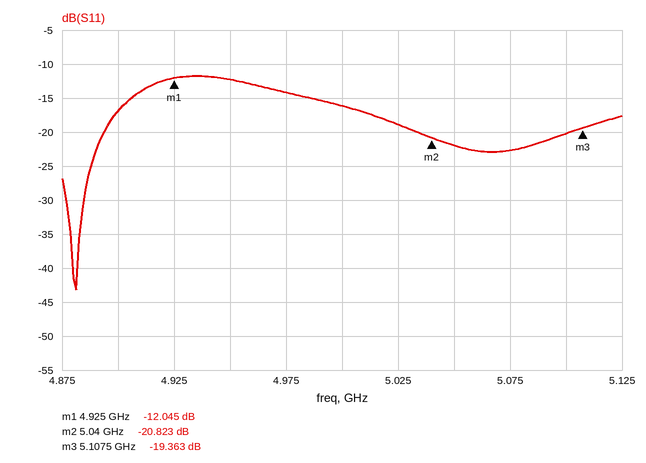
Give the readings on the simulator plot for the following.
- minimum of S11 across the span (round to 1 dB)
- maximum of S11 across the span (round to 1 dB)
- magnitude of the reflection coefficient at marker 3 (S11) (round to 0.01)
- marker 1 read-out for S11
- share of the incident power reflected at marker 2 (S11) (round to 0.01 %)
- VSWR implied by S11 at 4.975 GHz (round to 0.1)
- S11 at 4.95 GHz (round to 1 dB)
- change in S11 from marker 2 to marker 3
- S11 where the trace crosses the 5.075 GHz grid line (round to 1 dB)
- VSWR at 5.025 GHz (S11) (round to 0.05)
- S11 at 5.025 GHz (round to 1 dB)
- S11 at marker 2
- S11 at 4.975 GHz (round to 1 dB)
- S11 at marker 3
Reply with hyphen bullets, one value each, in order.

- -43 dB
- -12 dB
- 0.11
- -12.045 dB
- 0.83 %
- 1.5
- -12 dB
- 1.460 dB
- -23 dB
- 1.25
- -19 dB
- -20.823 dB
- -14 dB
- -19.363 dB
